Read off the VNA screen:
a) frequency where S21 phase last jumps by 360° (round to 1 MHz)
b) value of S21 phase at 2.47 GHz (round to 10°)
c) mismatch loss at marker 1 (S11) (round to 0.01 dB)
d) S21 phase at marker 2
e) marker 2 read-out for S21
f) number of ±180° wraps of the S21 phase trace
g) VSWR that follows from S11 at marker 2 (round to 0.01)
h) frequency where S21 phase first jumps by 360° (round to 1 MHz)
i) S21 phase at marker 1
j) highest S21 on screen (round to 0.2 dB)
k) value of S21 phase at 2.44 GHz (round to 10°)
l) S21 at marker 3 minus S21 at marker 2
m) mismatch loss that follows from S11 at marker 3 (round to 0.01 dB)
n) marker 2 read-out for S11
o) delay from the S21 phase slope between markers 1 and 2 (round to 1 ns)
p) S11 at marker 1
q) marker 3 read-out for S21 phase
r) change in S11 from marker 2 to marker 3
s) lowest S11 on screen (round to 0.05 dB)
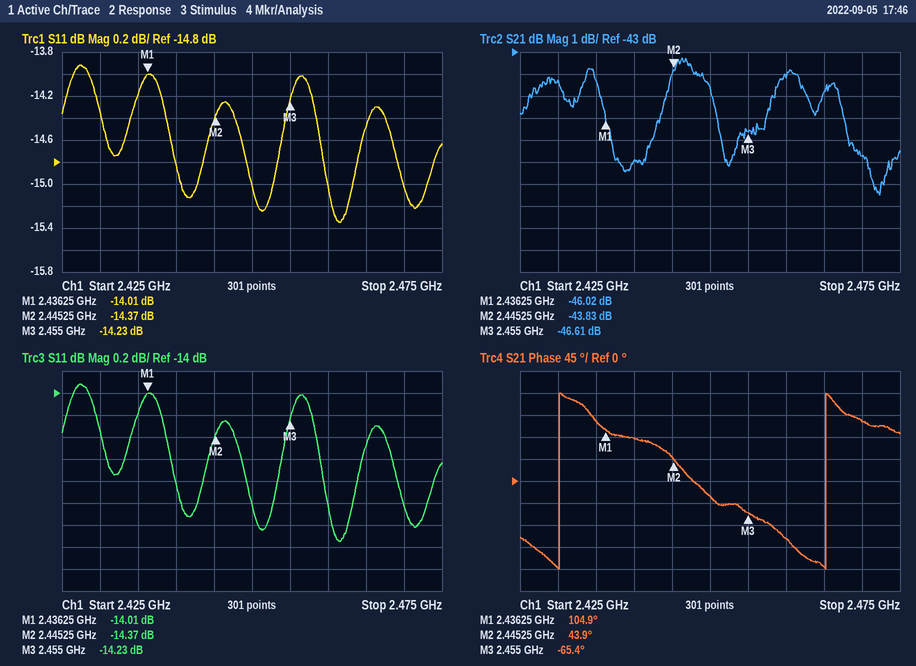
2.465 GHz
120°
0.18 dB
43.9°
-43.83 dB
2
1.47
2.430 GHz
104.9°
-43.2 dB
90°
-2.78 dB
0.17 dB
-14.37 dB
19 ns
-14.01 dB
-65.4°
0.14 dB
-15.35 dB
